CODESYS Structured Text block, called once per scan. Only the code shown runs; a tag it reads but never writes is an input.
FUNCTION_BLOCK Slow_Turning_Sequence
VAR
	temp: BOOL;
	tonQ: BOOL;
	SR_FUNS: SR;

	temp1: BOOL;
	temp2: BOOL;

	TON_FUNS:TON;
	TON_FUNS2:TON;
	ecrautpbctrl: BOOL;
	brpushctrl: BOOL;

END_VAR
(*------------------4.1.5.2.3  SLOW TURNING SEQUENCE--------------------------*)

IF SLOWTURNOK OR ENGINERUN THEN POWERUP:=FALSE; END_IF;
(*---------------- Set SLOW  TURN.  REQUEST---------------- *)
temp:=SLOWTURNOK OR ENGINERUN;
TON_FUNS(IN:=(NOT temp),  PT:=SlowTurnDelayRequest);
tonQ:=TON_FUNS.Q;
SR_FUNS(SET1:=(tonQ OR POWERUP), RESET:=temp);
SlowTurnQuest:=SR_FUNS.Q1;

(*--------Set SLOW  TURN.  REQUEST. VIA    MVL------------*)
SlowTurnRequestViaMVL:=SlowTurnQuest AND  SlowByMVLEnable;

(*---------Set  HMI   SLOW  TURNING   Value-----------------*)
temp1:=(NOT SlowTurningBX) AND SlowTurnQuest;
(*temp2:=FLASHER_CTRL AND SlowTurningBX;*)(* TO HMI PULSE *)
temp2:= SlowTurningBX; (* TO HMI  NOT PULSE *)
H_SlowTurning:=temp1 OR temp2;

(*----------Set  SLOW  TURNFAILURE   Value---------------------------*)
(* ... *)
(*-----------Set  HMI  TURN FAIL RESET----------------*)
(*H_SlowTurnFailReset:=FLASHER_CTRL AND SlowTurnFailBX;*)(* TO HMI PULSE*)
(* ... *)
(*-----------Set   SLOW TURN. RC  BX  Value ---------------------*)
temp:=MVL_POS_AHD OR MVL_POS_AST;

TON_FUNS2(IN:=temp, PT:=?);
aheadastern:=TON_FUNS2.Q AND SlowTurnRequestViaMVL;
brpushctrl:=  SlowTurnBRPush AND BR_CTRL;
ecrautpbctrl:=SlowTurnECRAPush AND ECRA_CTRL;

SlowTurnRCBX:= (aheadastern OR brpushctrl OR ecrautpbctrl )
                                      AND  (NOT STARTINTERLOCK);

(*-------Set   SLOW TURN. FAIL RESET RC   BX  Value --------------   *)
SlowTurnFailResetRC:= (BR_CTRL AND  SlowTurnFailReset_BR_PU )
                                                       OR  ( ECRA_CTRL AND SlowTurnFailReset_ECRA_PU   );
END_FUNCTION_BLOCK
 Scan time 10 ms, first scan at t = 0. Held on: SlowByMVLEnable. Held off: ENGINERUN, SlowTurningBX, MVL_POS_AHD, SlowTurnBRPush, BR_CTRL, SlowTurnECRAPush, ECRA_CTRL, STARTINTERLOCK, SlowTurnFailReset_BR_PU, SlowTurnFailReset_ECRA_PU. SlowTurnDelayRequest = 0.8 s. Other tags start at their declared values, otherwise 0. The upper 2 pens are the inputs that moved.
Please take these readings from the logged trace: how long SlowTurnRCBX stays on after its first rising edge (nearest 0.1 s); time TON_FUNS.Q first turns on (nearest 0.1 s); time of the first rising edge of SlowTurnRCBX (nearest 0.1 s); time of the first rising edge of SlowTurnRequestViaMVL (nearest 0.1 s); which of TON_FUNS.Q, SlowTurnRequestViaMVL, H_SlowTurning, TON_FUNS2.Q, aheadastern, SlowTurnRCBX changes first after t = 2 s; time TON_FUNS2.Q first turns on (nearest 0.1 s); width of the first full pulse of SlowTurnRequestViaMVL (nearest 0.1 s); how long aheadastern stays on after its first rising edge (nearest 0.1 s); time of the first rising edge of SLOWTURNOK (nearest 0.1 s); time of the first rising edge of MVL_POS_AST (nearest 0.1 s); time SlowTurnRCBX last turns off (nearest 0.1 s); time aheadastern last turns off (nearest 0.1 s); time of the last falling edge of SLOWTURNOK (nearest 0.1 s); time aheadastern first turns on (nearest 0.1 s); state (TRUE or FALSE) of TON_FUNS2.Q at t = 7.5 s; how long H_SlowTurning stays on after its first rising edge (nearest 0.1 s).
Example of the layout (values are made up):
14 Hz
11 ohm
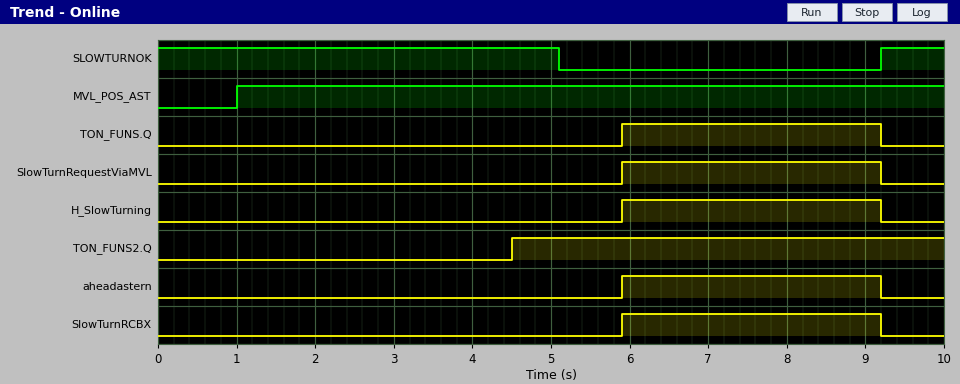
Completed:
3.3 s
5.9 s
5.9 s
5.9 s
TON_FUNS2.Q
4.5 s
3.3 s
3.3 s
9.2 s
1.0 s
9.2 s
9.2 s
5.1 s
5.9 s
TRUE
3.3 s
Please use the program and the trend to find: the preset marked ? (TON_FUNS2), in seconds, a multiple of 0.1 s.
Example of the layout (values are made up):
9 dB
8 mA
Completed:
3.5 s
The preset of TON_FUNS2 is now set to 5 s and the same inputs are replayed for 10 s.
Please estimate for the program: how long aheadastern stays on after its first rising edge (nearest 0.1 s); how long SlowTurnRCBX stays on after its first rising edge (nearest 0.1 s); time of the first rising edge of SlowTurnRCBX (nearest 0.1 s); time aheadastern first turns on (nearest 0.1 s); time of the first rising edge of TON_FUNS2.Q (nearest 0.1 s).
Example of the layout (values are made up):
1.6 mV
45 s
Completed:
3.2 s
3.2 s
6.0 s
6.0 s
6.0 s
